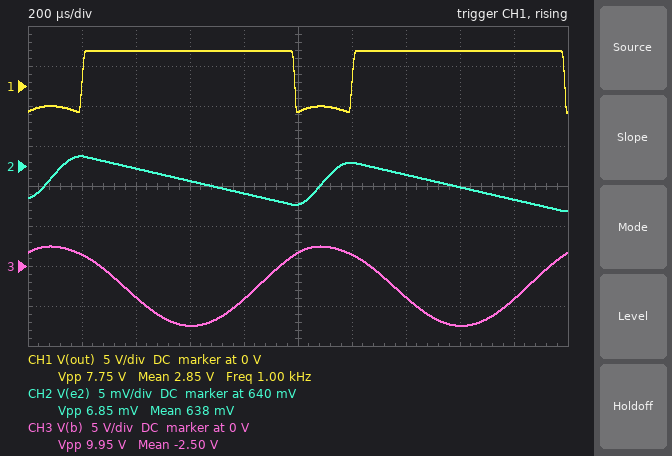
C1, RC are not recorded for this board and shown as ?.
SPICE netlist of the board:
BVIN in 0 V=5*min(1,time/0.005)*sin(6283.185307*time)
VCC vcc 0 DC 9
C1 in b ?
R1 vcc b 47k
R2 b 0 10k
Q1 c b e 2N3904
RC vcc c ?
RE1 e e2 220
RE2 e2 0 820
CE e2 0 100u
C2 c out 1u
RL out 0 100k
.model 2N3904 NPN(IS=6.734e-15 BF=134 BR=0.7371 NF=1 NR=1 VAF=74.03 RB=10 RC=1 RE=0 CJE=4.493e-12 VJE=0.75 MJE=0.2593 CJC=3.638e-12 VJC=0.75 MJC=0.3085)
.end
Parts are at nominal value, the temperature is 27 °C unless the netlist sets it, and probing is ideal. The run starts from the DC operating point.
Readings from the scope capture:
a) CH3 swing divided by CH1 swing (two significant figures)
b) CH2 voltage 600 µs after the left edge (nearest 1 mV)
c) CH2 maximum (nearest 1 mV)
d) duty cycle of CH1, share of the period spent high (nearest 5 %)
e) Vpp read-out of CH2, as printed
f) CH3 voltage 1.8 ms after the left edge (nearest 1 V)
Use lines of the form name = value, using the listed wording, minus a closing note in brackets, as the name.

CH3 swing divided by CH1 swing = 1.3
CH2 voltage 600 µs after the left edge = 638 mV
CH2 maximum = 641 mV
duty cycle of CH1, share of the period spent high = 80 %
Vpp read-out of CH2, as printed = 6.85 mV
CH3 voltage 1.8 ms after the left edge = -4 V
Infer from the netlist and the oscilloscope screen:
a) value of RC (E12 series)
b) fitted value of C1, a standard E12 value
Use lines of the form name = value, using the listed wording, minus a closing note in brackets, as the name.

value of RC = 8.2 kΩ
fitted value of C1, a standard E12 value = 680 nF
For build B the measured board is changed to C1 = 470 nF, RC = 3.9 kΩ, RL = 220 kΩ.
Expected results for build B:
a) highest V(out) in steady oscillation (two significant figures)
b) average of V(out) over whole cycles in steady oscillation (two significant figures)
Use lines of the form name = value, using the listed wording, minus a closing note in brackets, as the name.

highest V(out) in steady oscillation = 2.9 V
average of V(out) over whole cycles in steady oscillation = 1.2 V
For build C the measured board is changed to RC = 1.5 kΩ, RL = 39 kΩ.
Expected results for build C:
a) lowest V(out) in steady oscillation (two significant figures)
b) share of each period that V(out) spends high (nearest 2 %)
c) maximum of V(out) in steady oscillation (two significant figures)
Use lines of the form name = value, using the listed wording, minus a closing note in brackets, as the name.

lowest V(out) in steady oscillation = -5.4 V
share of each period that V(out) spends high = 76 %
maximum of V(out) in steady oscillation = 1.5 V
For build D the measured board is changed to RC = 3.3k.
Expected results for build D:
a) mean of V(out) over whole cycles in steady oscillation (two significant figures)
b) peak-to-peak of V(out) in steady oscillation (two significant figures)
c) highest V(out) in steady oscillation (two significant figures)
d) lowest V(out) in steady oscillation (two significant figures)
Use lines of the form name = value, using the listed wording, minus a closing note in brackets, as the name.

mean of V(out) over whole cycles in steady oscillation = 650 mV
peak-to-peak of V(out) in steady oscillation = 7.6 V
highest V(out) in steady oscillation = 2.2 V
lowest V(out) in steady oscillation = -5.3 V
